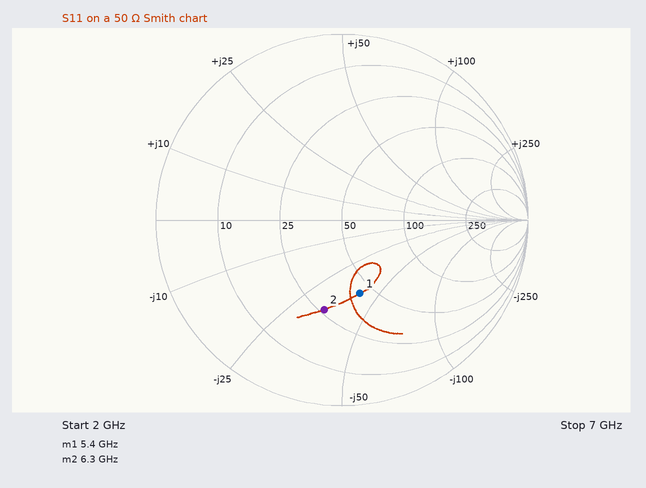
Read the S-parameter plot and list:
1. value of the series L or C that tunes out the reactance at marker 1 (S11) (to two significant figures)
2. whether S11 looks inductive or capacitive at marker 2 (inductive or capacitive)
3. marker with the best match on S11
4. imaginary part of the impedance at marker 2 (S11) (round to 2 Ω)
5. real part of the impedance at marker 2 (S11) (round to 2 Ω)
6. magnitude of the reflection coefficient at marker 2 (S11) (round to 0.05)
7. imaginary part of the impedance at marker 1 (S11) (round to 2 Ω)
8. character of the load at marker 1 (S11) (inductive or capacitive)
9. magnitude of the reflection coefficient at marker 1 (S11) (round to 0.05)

1.2 nH
capacitive
marker 1
-34 Ω
26 Ω
0.50
-40 Ω
capacitive
0.40
